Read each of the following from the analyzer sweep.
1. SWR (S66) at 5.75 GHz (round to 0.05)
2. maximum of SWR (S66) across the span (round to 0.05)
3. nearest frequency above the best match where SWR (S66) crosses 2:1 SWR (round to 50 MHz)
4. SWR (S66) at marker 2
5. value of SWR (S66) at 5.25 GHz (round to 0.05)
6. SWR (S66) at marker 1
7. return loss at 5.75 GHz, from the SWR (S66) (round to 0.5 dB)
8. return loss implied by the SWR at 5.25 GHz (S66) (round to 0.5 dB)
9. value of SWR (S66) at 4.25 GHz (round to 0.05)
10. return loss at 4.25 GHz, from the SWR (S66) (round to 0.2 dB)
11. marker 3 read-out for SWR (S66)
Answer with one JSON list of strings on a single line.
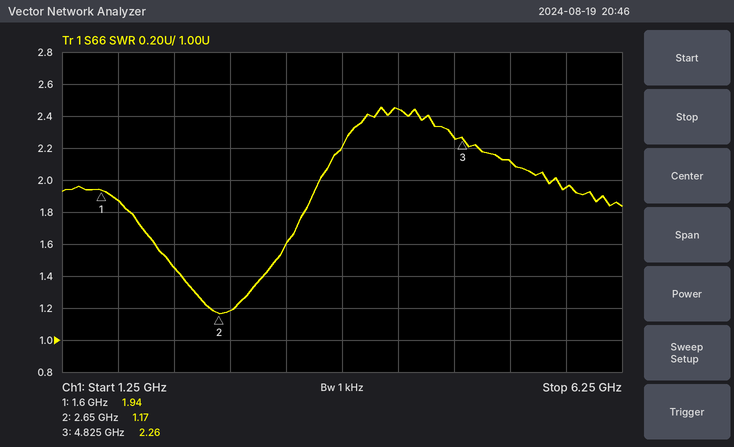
["1.95", "2.45", "3.55 GHz", "1.17", "2.10", "1.94", "10.0 dB", "9.0 dB", "2.45", "7.6 dB", "2.26"]
